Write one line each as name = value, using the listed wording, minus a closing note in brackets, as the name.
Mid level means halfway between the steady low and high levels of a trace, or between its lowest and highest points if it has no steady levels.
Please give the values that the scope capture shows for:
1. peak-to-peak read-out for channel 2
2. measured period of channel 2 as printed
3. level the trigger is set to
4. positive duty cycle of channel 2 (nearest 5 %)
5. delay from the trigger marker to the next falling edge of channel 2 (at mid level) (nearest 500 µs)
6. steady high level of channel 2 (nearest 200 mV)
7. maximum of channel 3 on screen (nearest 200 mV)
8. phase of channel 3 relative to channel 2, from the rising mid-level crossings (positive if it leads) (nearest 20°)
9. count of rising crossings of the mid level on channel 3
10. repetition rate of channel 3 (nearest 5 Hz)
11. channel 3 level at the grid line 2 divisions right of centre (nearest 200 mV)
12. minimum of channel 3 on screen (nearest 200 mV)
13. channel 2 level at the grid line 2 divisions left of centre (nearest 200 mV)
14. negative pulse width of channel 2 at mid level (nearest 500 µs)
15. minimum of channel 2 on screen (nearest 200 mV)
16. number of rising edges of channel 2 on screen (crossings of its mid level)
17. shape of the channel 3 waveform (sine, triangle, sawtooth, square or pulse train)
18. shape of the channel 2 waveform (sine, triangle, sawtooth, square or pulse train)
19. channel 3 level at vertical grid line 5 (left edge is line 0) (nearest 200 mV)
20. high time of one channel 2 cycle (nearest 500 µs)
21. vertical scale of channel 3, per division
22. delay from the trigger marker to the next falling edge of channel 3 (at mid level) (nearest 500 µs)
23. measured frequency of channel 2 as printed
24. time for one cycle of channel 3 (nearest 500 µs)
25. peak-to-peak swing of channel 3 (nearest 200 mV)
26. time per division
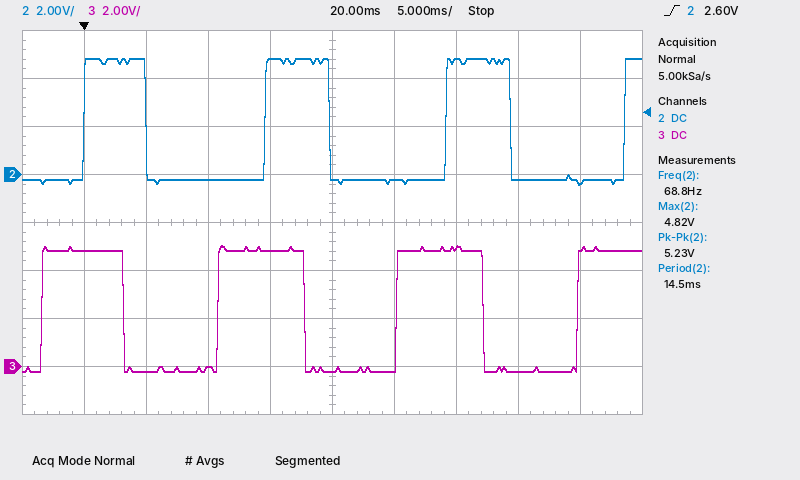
peak-to-peak read-out for channel 2 = 5.23 V
measured period of channel 2 as printed = 14.5 ms
level the trigger is set to = 2.60 V
positive duty cycle of channel 2 = 35 %
delay from the trigger marker to the next falling edge of channel 2 (at mid level) = 5.0 ms
steady high level of channel 2 = 4.8 V
maximum of channel 3 on screen = 5.0 V
phase of channel 3 relative to channel 2, from the rising mid-level crossings (positive if it leads) = +100°
count of rising crossings of the mid level on channel 3 = 4
repetition rate of channel 3 = 70 Hz
channel 3 level at the grid line 2 divisions right of centre = 5.0 V
minimum of channel 3 on screen = -200 mV
channel 2 level at the grid line 2 divisions left of centre = -200 mV
negative pulse width of channel 2 at mid level = 9.5 ms
minimum of channel 2 on screen = -400 mV
number of rising edges of channel 2 on screen = 4
shape of the channel 3 waveform = square
shape of the channel 2 waveform = pulse train
channel 3 level at vertical grid line 5 (left edge is line 0) = -200 mV
high time of one channel 2 cycle = 5.0 ms
vertical scale of channel 3, per division = 2 V
delay from the trigger marker to the next falling edge of channel 3 (at mid level) = 3.0 ms
measured frequency of channel 2 as printed = 68.8 Hz
time for one cycle of channel 3 = 14.5 ms
peak-to-peak swing of channel 3 = 5.2 V
time per division = 5 ms
